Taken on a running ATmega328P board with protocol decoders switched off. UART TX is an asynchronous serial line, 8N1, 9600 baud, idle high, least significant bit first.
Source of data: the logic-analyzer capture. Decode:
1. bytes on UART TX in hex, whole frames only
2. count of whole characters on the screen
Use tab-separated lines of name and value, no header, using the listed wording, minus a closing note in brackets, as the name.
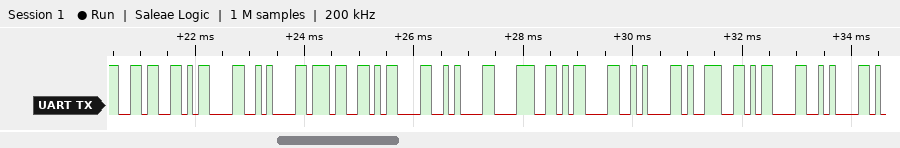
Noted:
bytes on UART TX in hex, whole frames only	0x36 0x0D 0x0A 0x37 0x0D 0x0A 0x38 0x0D 0x0A 0x39 0x0D 0x0A
count of whole characters on the screen	12
